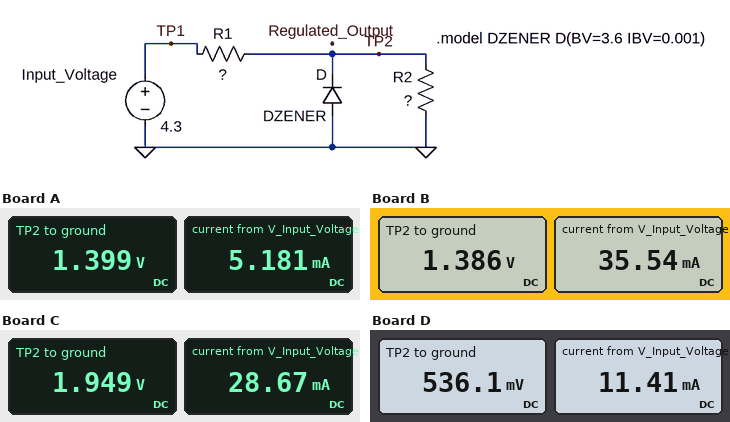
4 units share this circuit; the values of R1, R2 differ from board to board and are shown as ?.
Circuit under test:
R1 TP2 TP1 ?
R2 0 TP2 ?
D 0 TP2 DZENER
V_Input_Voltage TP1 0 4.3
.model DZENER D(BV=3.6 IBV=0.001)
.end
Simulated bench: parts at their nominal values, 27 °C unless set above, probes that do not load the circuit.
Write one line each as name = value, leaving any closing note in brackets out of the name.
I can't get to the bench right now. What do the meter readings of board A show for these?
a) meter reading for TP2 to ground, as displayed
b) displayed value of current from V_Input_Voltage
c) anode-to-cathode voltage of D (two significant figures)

meter reading for TP2 to ground, as displayed = 1.399 V
displayed value of current from V_Input_Voltage = 5.181 mA
anode-to-cathode voltage of D = -1.4 V
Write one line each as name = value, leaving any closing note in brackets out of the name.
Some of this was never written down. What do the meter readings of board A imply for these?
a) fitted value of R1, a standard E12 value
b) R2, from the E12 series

fitted value of R1, a standard E12 value = 560 Ω
R2, from the E12 series = 270 Ω
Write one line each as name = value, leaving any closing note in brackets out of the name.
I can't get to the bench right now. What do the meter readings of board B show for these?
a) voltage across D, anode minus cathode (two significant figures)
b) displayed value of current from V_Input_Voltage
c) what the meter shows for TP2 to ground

voltage across D, anode minus cathode = -1.4 V
displayed value of current from V_Input_Voltage = 35.54 mA
what the meter shows for TP2 to ground = 1.386 V
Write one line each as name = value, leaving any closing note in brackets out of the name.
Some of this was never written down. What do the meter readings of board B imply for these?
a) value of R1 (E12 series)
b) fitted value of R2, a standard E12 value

value of R1 = 82 Ω
fitted value of R2, a standard E12 value = 39 Ω
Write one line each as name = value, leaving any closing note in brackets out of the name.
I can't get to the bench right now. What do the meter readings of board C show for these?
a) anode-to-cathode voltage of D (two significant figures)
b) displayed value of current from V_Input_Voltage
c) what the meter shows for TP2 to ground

anode-to-cathode voltage of D = -1.9 V
displayed value of current from V_Input_Voltage = 28.67 mA
what the meter shows for TP2 to ground = 1.949 V
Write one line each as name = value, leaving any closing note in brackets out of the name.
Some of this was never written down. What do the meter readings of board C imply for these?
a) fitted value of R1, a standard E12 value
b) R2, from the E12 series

fitted value of R1, a standard E12 value = 82 Ω
R2, from the E12 series = 68 Ω
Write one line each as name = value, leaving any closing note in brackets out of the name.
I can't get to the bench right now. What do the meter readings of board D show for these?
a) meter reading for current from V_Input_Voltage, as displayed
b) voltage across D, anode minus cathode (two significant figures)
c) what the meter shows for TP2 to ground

meter reading for current from V_Input_Voltage, as displayed = 11.41 mA
voltage across D, anode minus cathode = -540 mV
what the meter shows for TP2 to ground = 536.1 mV
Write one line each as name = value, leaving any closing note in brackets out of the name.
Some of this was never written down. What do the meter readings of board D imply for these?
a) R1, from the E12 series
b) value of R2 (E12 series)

R1, from the E12 series = 330 Ω
value of R2 = 47 Ω
